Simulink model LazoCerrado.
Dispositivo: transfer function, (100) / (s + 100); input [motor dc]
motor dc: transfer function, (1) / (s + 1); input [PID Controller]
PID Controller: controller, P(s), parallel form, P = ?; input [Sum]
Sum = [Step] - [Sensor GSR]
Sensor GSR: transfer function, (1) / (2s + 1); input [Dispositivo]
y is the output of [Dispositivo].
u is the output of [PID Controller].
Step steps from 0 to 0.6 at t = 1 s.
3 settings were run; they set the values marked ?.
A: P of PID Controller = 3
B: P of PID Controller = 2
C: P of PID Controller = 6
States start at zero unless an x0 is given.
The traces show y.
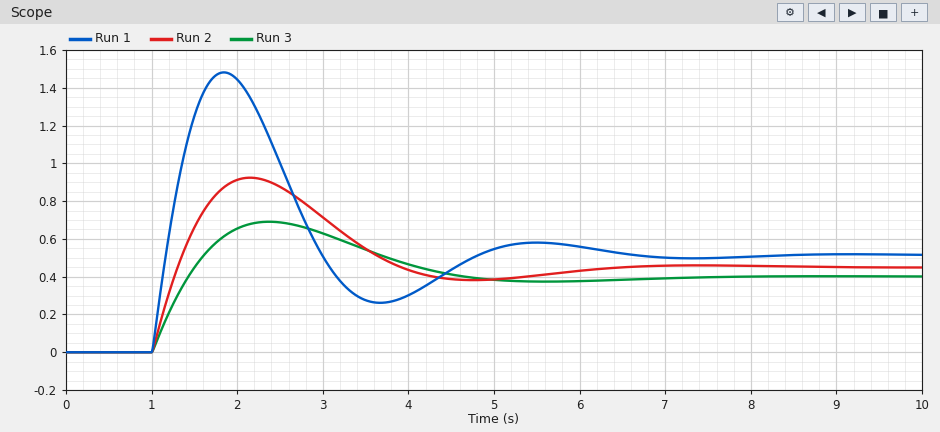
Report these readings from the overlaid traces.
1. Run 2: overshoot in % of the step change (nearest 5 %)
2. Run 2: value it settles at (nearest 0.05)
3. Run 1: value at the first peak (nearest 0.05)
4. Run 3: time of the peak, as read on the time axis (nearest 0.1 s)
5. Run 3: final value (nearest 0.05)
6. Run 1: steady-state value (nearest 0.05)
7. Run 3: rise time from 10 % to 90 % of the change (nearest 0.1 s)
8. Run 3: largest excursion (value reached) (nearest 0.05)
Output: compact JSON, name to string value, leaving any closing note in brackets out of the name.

{"Run 2: overshoot in % of the step change": "105 %", "Run 2: value it settles at": "0.45", "Run 1: value at the first peak": "1.50", "Run 3: time of the peak, as read on the time axis": "2.4 s", "Run 3: final value": "0.40", "Run 1: steady-state value": "0.50", "Run 3: rise time from 10 % to 90 % of the change": "0.3 s", "Run 3: largest excursion (value reached)": "0.70"}
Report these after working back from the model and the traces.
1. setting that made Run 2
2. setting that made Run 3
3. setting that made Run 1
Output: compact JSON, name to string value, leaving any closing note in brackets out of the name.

{"setting that made Run 2": "A", "setting that made Run 3": "B", "setting that made Run 1": "C"}
